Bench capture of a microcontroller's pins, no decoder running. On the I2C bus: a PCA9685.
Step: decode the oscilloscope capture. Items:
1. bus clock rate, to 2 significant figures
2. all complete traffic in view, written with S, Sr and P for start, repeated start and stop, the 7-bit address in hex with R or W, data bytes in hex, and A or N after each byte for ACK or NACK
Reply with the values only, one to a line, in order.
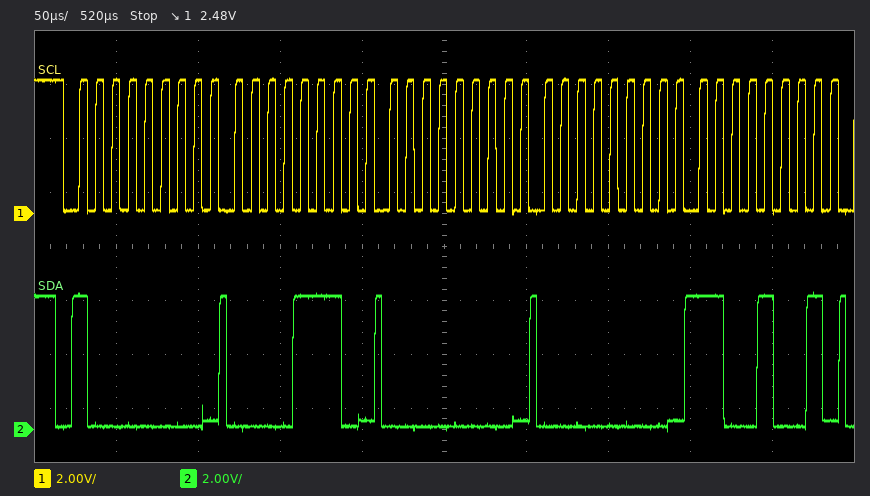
100 kHz
S 40W A 0E A 00 A 00 A C9 A
